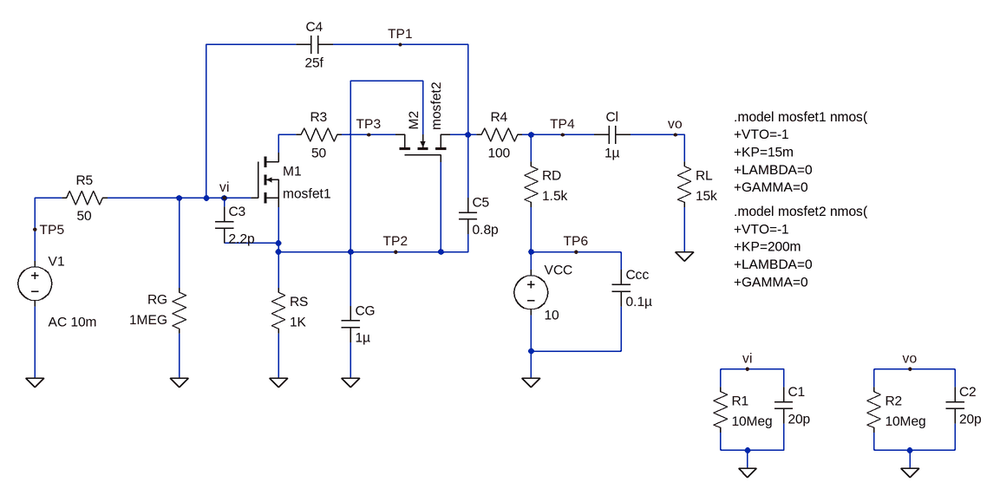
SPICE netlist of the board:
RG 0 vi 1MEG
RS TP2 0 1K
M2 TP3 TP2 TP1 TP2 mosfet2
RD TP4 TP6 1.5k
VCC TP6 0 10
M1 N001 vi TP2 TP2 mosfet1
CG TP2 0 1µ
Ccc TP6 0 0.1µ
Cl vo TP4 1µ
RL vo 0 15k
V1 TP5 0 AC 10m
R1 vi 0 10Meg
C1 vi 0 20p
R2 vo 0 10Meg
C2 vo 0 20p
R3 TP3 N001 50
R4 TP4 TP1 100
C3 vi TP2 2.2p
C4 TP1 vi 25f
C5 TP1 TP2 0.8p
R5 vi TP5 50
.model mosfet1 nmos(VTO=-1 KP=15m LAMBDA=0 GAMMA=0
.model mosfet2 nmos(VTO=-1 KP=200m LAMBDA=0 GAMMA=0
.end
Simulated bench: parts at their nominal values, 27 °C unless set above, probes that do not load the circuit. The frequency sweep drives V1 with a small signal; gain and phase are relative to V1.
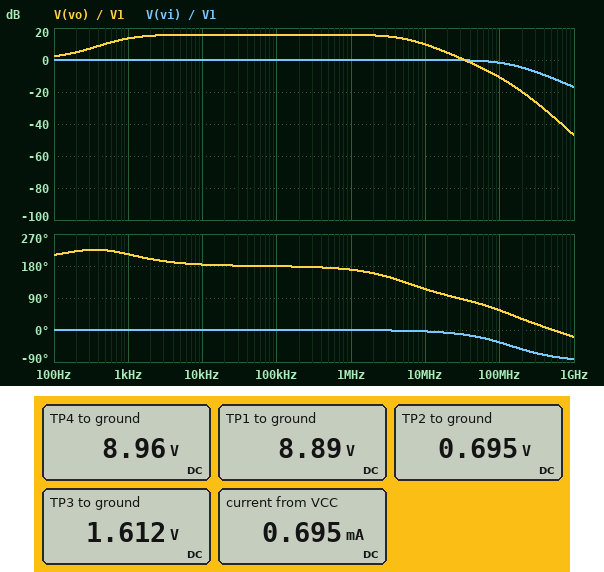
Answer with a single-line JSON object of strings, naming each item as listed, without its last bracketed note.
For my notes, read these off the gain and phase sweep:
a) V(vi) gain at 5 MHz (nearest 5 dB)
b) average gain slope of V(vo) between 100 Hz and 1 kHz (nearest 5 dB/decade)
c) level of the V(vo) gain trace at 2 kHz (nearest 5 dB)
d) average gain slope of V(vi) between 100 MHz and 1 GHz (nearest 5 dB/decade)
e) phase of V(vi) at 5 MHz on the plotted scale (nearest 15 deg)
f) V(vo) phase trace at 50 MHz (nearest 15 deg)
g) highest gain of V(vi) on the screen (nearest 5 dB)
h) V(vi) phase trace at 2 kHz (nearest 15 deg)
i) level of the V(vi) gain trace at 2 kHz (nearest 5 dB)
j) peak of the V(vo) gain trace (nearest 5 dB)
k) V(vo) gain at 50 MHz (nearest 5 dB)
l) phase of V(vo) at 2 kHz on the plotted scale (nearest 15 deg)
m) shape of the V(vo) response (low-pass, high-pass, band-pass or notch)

{"V(vi) gain at 5 MHz": "0 dB", "average gain slope of V(vo) between 100 Hz and 1 kHz": "10 dB/decade", "level of the V(vo) gain trace at 2 kHz": "15 dB", "average gain slope of V(vi) between 100 MHz and 1 GHz": "-15 dB/decade", "phase of V(vi) at 5 MHz on the plotted scale": "0 deg", "V(vo) phase trace at 50 MHz": "75 deg", "highest gain of V(vi) on the screen": "0 dB", "V(vi) phase trace at 2 kHz": "0 deg", "level of the V(vi) gain trace at 2 kHz": "0 dB", "peak of the V(vo) gain trace": "15 dB", "V(vo) gain at 50 MHz": "-5 dB", "phase of V(vo) at 2 kHz on the plotted scale": "195 deg", "shape of the V(vo) response": "band-pass"}
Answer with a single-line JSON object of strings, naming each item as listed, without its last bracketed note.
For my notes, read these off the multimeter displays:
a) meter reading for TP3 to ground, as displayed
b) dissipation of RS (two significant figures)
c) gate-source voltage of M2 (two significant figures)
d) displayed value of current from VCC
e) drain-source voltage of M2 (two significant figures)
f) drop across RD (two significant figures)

{"meter reading for TP3 to ground, as displayed": "1.612 V", "dissipation of RS": "480 µW", "gate-source voltage of M2": "-8.2 V", "displayed value of current from VCC": "0.695 mA", "drain-source voltage of M2": "-7.3 V", "drop across RD": "1.0 V"}
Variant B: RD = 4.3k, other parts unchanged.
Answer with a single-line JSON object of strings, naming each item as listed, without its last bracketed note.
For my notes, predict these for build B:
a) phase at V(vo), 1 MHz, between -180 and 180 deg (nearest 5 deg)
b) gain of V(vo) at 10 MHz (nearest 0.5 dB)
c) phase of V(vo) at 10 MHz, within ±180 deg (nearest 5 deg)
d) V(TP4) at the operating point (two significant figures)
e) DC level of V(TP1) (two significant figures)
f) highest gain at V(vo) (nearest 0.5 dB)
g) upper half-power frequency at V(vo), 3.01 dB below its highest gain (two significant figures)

{"phase at V(vo), 1 MHz, between -180 and 180 deg": "155 deg", "gain of V(vo) at 10 MHz": "10.5 dB", "phase of V(vo) at 10 MHz, within ±180 deg": "100 deg", "V(TP4) at the operating point": "7.0 V", "DC level of V(TP1)": "6.9 V", "highest gain at V(vo)": "23.5 dB", "upper half-power frequency at V(vo), 3.01 dB below its highest gain": "2.3 MHz"}
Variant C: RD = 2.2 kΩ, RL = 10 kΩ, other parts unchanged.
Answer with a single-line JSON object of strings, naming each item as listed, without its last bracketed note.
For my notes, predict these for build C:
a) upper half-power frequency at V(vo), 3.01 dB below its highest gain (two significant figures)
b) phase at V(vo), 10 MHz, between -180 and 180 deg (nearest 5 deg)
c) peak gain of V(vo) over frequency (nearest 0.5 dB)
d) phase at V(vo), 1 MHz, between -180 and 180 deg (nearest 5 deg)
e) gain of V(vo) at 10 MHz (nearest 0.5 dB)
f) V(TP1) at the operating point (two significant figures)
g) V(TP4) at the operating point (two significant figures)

{"upper half-power frequency at V(vo), 3.01 dB below its highest gain": "4.2 MHz", "phase at V(vo), 10 MHz, between -180 and 180 deg": "110 deg", "peak gain of V(vo) over frequency": "18.5 dB", "phase at V(vo), 1 MHz, between -180 and 180 deg": "165 deg", "gain of V(vo) at 10 MHz": "10.0 dB", "V(TP1) at the operating point": "8.4 V", "V(TP4) at the operating point": "8.5 V"}
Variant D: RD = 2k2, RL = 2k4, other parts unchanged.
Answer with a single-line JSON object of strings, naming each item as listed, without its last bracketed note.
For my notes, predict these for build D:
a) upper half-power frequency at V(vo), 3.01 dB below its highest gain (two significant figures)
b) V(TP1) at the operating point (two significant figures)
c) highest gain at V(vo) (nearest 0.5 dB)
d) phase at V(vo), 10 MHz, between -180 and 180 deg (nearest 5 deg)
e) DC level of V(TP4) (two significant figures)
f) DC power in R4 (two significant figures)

{"upper half-power frequency at V(vo), 3.01 dB below its highest gain": "6.6 MHz", "V(TP1) at the operating point": "8.4 V", "highest gain at V(vo)": "14.5 dB", "phase at V(vo), 10 MHz, between -180 and 180 deg": "120 deg", "DC level of V(TP4)": "8.5 V", "DC power in R4": "48 µW"}
